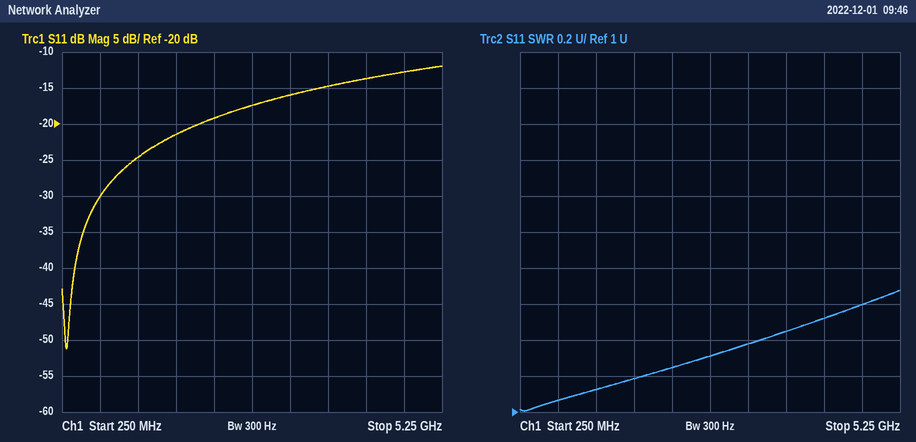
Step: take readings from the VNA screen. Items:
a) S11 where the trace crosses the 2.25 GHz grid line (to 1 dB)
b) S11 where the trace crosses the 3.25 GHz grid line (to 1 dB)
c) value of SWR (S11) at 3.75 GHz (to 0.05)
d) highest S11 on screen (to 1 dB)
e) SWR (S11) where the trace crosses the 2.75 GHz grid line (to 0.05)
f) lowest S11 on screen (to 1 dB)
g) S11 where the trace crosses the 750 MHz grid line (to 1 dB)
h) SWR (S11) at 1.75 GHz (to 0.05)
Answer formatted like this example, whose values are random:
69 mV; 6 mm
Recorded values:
-19 dB; -16 dB; 1.45; -12 dB; 1.30; -51 dB; -30 dB; 1.20
